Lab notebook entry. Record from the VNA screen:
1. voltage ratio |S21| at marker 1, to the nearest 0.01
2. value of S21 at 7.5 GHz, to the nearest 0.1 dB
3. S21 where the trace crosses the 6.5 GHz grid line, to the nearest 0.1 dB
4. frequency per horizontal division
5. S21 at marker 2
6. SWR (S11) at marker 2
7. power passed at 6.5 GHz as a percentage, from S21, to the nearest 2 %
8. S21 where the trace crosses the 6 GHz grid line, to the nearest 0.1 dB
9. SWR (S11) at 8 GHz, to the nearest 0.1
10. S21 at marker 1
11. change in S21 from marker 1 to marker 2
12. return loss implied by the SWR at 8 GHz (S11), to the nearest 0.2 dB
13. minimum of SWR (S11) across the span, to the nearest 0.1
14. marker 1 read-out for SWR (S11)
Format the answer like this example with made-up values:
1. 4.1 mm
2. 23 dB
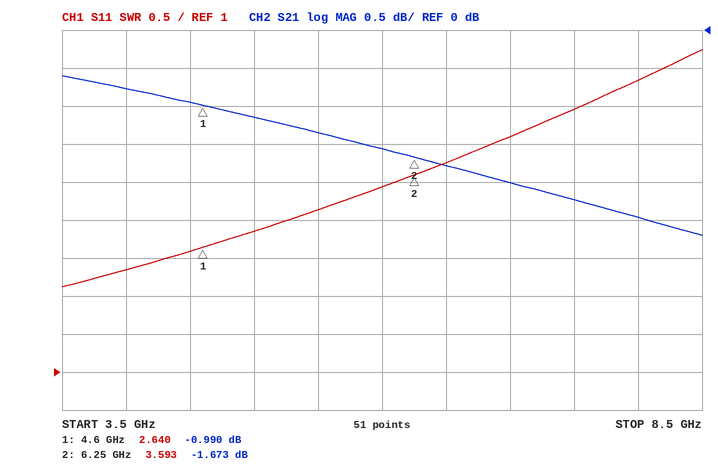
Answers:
1. 0.89
2. -2.2 dB
3. -1.8 dB
4. 500 MHz
5. -1.673 dB
6. 3.593
7. 66 %
8. -1.6 dB
9. 4.8
10. -0.990 dB
11. -0.683 dB
12. 3.6 dB
13. 2.1
14. 2.640
